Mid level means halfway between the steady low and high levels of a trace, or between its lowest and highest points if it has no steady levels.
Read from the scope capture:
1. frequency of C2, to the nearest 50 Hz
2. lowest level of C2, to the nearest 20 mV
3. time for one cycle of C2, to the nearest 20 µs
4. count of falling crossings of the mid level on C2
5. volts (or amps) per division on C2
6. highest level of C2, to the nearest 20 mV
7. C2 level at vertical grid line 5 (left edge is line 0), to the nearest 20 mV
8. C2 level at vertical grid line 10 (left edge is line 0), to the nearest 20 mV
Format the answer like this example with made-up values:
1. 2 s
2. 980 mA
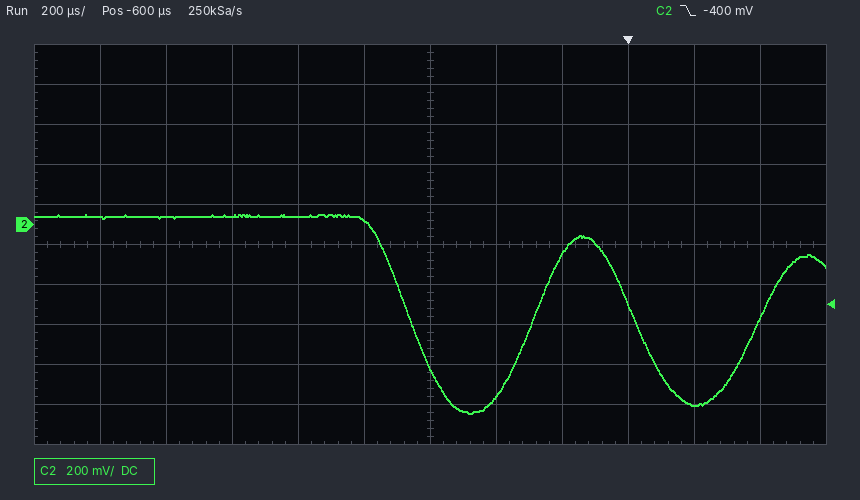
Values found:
1. 1.45 kHz
2. -940 mV
3. 680 µs
4. 2
5. 200 mV
6. 40 mV
7. 20 mV
8. -900 mV
